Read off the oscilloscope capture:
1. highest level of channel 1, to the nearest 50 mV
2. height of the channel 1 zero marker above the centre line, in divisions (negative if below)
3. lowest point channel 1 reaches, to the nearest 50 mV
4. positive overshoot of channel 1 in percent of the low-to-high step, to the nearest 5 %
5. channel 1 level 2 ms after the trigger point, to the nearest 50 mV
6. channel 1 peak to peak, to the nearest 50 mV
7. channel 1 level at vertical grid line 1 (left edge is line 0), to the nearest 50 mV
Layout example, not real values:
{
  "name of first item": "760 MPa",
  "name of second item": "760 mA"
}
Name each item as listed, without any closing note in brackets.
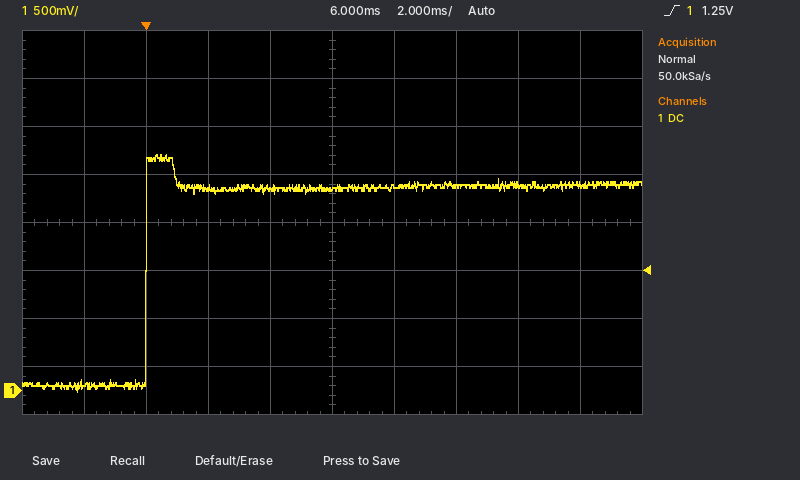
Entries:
{
  "highest level of channel 1, to the nearest 50 mV": "2.45 V",
  "height of the channel 1 zero marker above the centre line, in divisions": "-3.5 div",
  "lowest point channel 1 reaches, to the nearest 50 mV": "0 mV",
  "positive overshoot of channel 1 in percent of the low-to-high step, to the nearest 5 %": "15 %",
  "channel 1 level 2 ms after the trigger point, to the nearest 50 mV": "2.10 V",
  "channel 1 peak to peak, to the nearest 50 mV": "2.45 V",
  "channel 1 level at vertical grid line 1 (left edge is line 0), to the nearest 50 mV": "50 mV"
}
